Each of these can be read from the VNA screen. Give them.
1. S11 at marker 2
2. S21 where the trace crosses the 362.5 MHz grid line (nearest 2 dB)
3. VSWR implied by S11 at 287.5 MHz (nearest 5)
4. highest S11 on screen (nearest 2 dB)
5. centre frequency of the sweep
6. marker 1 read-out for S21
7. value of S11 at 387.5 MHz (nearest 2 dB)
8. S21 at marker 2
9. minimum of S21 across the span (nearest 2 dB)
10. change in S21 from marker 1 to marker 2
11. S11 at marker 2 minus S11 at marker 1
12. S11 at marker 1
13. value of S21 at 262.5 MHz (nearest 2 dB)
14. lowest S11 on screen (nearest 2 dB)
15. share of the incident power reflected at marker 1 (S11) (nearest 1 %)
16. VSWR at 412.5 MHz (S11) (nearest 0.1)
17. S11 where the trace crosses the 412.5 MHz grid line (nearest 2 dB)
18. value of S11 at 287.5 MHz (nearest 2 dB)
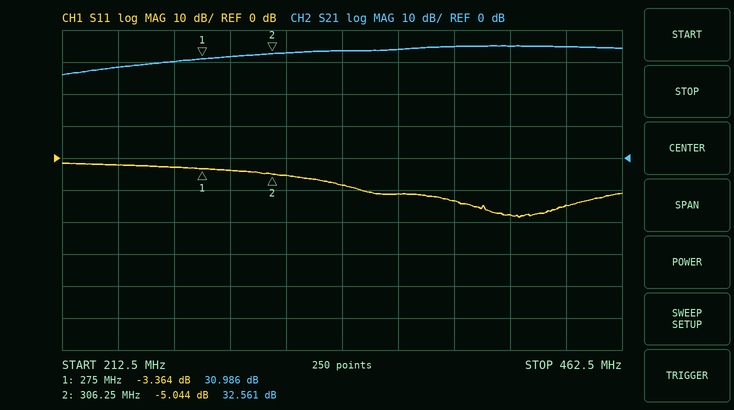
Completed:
-5.044 dB
34 dB
5
-2 dB
337.5 MHz
30.986 dB
-14 dB
32.561 dB
26 dB
1.575 dB
-1.680 dB
-3.364 dB
30 dB
-18 dB
46 %
1.3
-18 dB
-4 dB
